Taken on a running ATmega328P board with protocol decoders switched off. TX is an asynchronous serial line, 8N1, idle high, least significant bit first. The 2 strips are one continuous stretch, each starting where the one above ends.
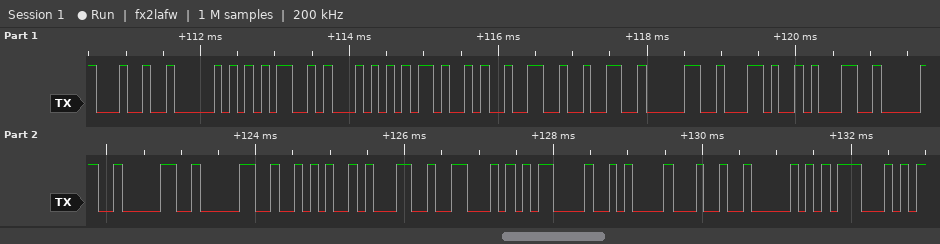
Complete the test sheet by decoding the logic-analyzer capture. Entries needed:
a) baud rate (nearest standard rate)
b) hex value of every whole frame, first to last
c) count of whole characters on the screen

9600 baud
0x24 0x50 0x4D 0x54 0x4B 0x32 0x32 0x30 0x2C 0x31 0x30 0x30 0x30 0x2A 0x31 0x46 0x0D 0x0A 0x24 0x50 0x47
21
